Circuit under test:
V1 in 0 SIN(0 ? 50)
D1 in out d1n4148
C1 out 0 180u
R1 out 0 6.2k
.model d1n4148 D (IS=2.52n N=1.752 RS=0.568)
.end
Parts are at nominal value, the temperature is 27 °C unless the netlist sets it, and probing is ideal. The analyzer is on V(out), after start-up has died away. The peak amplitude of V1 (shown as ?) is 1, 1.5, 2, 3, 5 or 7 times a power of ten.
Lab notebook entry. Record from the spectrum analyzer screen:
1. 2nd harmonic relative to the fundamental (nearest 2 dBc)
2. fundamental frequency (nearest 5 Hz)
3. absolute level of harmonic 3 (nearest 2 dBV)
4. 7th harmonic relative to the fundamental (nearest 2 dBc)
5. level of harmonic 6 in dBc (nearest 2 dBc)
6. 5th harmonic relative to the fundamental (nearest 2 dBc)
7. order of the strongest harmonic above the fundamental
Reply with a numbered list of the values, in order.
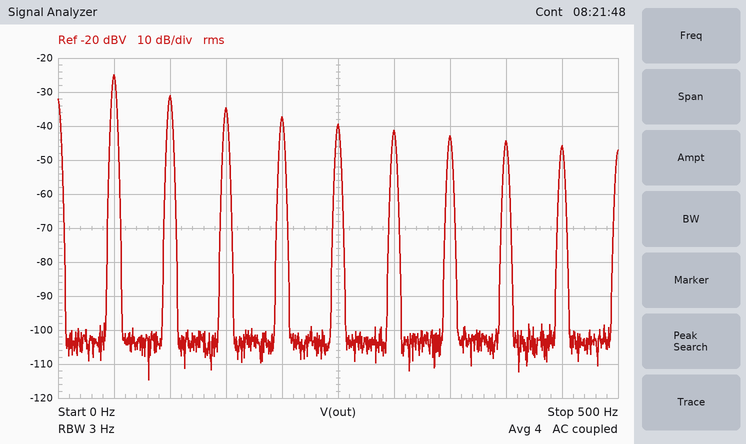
1. -6 dBc
2. 50 Hz
3. -34 dBV
4. -18 dBc
5. -16 dBc
6. -14 dBc
7. 2
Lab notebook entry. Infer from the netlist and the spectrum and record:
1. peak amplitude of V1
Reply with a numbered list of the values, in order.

1. 15 V
